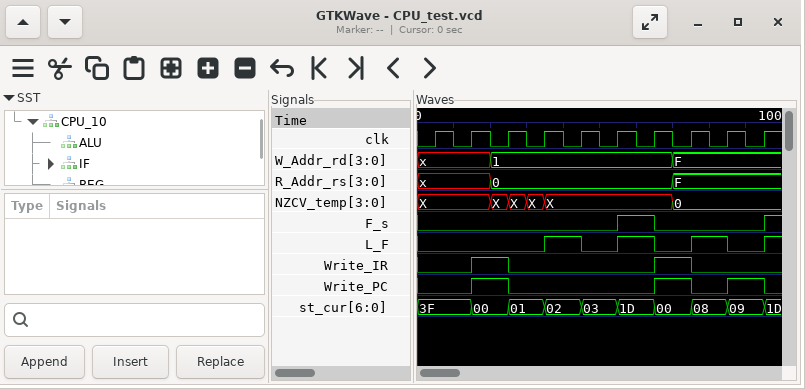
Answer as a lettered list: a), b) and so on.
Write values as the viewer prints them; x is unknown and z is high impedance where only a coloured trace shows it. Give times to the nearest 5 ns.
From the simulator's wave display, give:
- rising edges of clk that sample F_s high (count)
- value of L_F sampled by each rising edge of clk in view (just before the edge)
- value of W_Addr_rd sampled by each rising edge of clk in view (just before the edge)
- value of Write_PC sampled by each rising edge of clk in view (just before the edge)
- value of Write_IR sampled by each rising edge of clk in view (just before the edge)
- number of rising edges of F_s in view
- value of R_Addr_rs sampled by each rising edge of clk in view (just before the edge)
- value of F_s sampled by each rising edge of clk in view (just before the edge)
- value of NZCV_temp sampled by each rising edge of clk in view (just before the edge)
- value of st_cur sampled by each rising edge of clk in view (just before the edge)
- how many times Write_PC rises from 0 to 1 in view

a) 1
b) 0 0 0 0 1 0 1 0 1 0
c) x, x, 1, 1, 1, 1, 1, F, F, F
d) 0 0 1 0 0 0 0 1 0 1
e) 0 0 1 0 0 0 0 1 0 0
f) 2
g) x, x, 0, 0, 0, 0, 0, F, F, F
h) 0 0 0 0 0 0 1 0 0 0
i) X, X, X, X, X, X, X, 0, 0, 0
j) 3F, 3F, 00, 01, 02, 03, 1D, 00, 08, 09
k) 3
